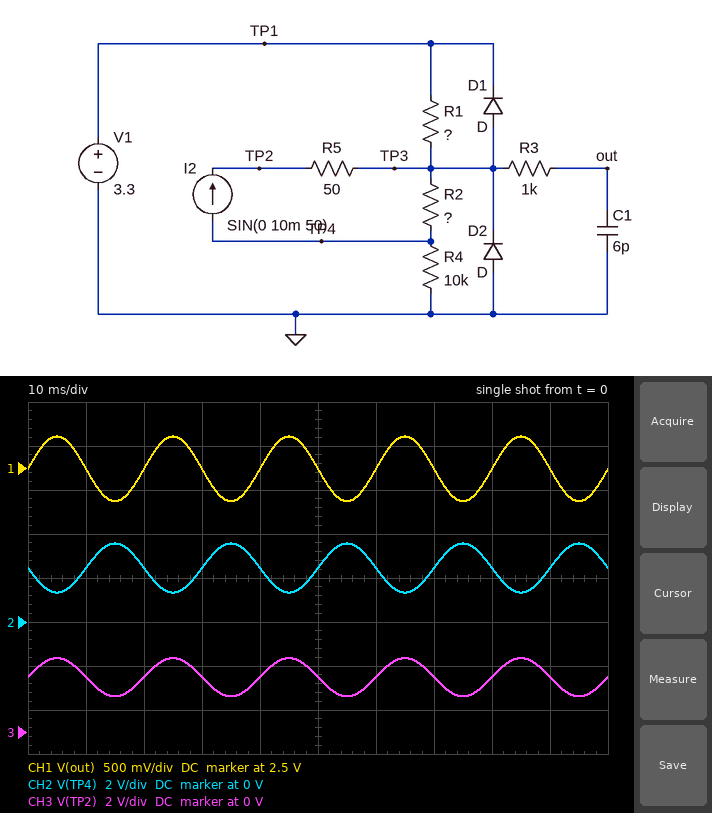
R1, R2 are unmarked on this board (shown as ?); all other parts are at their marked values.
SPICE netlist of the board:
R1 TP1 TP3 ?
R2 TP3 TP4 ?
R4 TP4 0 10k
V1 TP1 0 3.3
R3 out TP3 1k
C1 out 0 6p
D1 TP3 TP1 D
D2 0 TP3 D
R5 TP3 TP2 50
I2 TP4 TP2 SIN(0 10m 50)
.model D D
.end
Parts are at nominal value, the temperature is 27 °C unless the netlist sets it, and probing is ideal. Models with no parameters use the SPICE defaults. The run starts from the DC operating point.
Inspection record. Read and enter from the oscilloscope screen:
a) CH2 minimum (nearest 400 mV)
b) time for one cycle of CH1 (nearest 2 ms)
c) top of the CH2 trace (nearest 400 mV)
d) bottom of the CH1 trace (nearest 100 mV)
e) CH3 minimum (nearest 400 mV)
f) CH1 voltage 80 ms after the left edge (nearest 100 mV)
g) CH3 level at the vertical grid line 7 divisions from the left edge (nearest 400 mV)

1.2 V
20 ms
3.6 V
2.1 V
1.6 V
2.5 V
2.4 V
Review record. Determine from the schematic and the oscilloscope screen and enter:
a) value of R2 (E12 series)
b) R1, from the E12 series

150 Ω
3.3 kΩ
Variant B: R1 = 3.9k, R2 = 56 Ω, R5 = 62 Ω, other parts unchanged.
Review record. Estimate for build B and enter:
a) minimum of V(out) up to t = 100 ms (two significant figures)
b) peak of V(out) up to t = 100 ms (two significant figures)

2.2 V
2.5 V
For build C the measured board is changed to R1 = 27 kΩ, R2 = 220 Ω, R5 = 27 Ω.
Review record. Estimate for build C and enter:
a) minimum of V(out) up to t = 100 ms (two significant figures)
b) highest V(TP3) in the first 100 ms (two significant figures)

-550 mV
2.5 V
